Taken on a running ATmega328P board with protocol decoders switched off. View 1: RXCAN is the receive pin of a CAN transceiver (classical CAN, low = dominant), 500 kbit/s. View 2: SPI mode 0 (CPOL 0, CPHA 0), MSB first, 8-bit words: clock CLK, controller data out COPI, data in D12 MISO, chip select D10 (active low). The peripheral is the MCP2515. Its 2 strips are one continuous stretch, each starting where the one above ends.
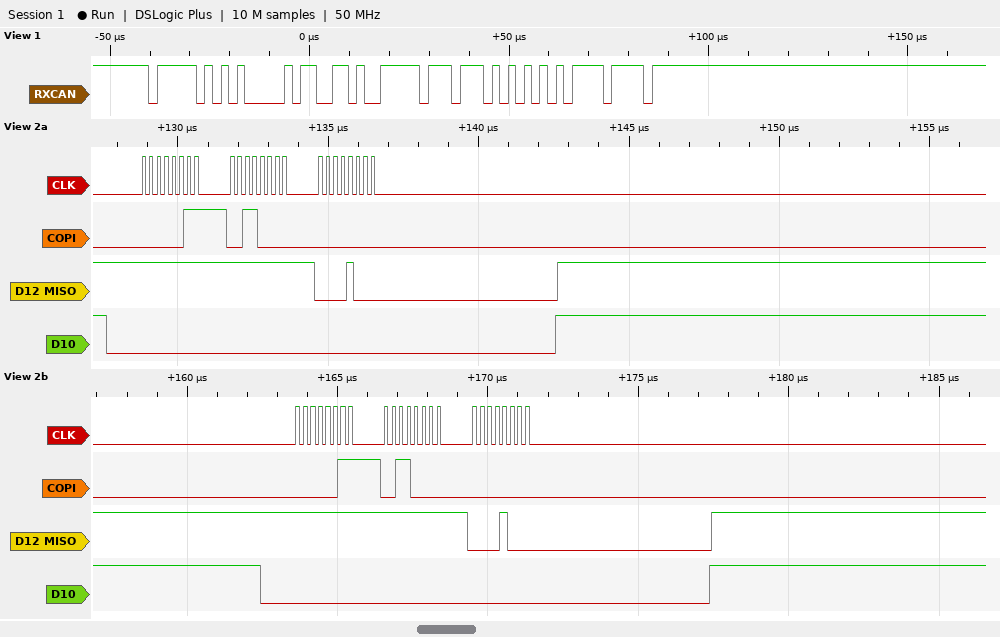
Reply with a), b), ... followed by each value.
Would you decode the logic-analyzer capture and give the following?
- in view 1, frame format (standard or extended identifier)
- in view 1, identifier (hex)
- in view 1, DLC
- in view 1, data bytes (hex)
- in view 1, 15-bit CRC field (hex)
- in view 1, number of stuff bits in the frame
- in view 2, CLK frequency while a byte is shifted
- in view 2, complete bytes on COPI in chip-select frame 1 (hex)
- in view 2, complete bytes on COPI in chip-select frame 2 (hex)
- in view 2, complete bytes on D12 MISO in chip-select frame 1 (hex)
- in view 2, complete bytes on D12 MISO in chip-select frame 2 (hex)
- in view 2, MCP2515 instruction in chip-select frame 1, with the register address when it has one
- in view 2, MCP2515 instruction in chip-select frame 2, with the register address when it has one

a) standard
b) 0x7EA
c) 3
d) 34 FF 75
e) 0x2AF7
f) 3
g) 4 MHz
h) 03 30 00
i) 03 30 00
j) FF FF 08
k) FF FF 08
l) READ 0x30
m) READ 0x30
